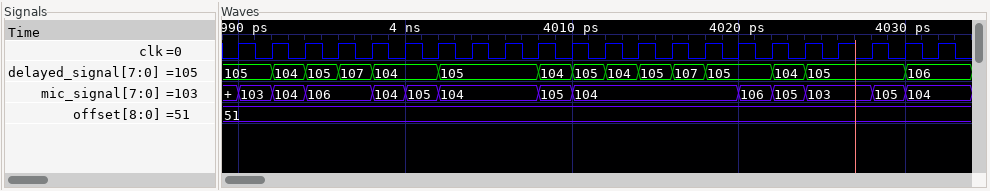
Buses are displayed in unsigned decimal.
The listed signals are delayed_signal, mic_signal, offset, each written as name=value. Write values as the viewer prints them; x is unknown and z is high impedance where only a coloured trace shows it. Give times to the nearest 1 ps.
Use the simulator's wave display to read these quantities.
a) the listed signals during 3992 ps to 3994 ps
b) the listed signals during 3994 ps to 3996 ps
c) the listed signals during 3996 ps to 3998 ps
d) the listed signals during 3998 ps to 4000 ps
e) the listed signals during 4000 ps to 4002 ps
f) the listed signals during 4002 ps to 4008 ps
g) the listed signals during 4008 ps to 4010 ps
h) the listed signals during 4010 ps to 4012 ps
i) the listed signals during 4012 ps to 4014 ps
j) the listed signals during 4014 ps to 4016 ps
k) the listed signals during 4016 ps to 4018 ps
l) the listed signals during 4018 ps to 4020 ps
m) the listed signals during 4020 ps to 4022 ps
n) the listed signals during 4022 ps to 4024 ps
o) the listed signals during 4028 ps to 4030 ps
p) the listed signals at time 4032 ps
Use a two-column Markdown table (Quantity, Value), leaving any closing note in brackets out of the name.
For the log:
| Quantity | Value |
|---|---|
| the listed signals during 3992 ps to 3994 ps | delayed_signal=104, mic_signal=104, offset=51 |
| the listed signals during 3994 ps to 3996 ps | delayed_signal=105, mic_signal=106, offset=51 |
| the listed signals during 3996 ps to 3998 ps | delayed_signal=107, mic_signal=106, offset=51 |
| the listed signals during 3998 ps to 4000 ps | delayed_signal=104, mic_signal=104, offset=51 |
| the listed signals during 4000 ps to 4002 ps | delayed_signal=104, mic_signal=105, offset=51 |
| the listed signals during 4002 ps to 4008 ps | delayed_signal=105, mic_signal=104, offset=51 |
| the listed signals during 4008 ps to 4010 ps | delayed_signal=104, mic_signal=105, offset=51 |
| the listed signals during 4010 ps to 4012 ps | delayed_signal=105, mic_signal=104, offset=51 |
| the listed signals during 4012 ps to 4014 ps | delayed_signal=104, mic_signal=104, offset=51 |
| the listed signals during 4014 ps to 4016 ps | delayed_signal=105, mic_signal=104, offset=51 |
| the listed signals during 4016 ps to 4018 ps | delayed_signal=107, mic_signal=104, offset=51 |
| the listed signals during 4018 ps to 4020 ps | delayed_signal=105, mic_signal=104, offset=51 |
| the listed signals during 4020 ps to 4022 ps | delayed_signal=105, mic_signal=106, offset=51 |
| the listed signals during 4022 ps to 4024 ps | delayed_signal=104, mic_signal=105, offset=51 |
| the listed signals during 4028 ps to 4030 ps | delayed_signal=105, mic_signal=105, offset=51 |
| the listed signals at time 4032 ps | delayed_signal=106, mic_signal=104, offset=51 |
